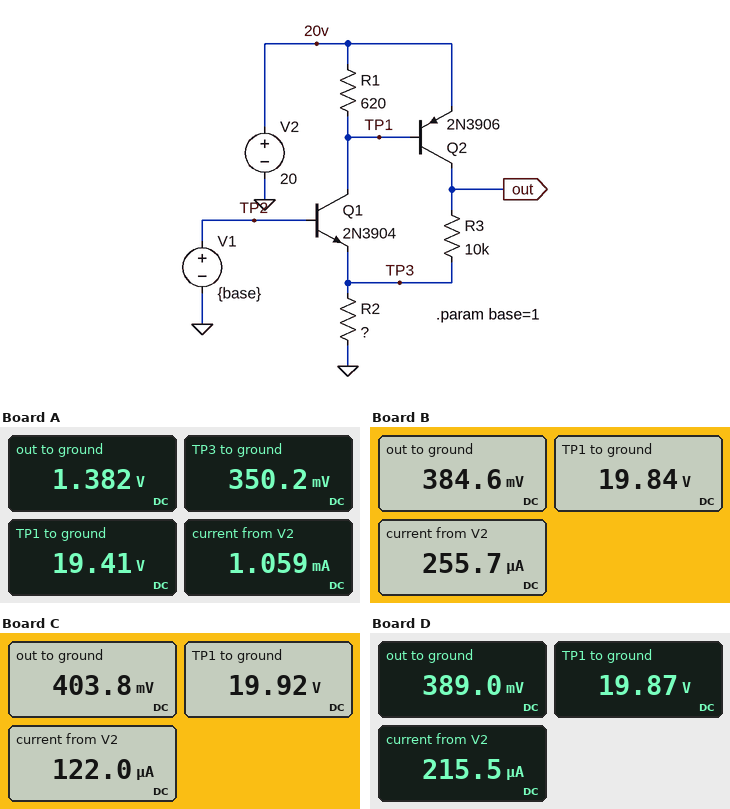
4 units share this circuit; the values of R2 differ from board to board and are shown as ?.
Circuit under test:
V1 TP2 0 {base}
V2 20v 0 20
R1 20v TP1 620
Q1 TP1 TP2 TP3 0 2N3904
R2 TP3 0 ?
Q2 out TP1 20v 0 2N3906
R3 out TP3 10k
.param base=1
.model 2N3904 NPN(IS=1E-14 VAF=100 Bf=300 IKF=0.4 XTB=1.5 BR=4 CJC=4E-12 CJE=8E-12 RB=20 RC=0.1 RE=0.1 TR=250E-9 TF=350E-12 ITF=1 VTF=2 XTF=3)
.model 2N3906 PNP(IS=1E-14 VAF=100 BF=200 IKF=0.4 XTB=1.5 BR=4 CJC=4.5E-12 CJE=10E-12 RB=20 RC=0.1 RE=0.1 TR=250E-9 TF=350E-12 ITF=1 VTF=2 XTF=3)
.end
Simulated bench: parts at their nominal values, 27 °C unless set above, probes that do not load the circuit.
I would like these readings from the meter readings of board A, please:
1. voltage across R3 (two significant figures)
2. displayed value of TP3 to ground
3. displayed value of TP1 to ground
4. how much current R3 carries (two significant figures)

1.0 V
350.2 mV
19.41 V
100 µA
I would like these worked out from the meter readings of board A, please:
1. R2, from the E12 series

330 Ω
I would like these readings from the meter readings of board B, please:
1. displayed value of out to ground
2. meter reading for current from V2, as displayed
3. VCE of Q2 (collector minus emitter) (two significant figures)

384.6 mV
255.7 µA
-20 V
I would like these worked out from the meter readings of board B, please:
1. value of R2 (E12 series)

1.5 kΩ
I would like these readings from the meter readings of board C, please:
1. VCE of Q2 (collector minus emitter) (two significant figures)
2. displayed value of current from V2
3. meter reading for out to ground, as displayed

-20 V
122.0 µA
403.8 mV
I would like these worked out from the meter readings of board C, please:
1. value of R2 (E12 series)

3.3 kΩ
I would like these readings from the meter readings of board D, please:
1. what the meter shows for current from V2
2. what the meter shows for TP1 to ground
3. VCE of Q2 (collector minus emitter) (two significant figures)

215.5 µA
19.87 V
-20 V
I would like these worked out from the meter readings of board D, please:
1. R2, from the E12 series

1.8 kΩ
